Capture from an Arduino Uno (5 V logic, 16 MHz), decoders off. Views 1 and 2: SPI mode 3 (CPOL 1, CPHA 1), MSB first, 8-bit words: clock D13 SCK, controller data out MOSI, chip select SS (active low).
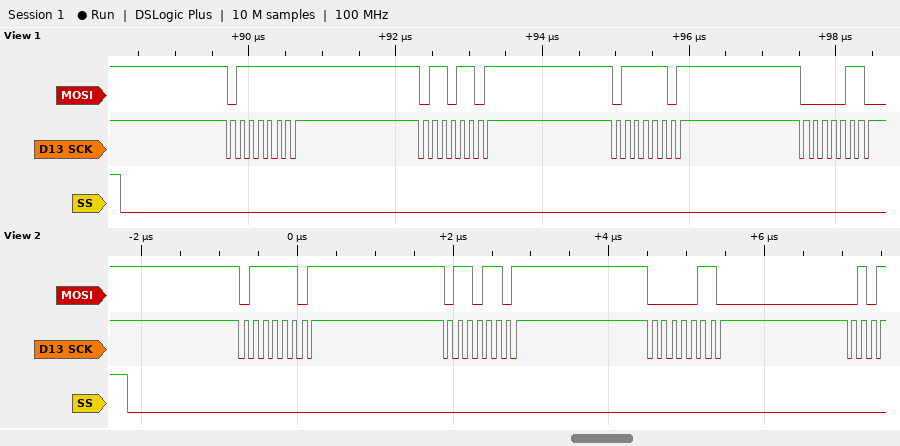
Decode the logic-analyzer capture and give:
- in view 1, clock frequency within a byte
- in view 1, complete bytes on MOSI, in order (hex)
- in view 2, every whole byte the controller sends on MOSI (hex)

8 MHz
7F 6D 7D 06
0x7D 0x6D 0x06
